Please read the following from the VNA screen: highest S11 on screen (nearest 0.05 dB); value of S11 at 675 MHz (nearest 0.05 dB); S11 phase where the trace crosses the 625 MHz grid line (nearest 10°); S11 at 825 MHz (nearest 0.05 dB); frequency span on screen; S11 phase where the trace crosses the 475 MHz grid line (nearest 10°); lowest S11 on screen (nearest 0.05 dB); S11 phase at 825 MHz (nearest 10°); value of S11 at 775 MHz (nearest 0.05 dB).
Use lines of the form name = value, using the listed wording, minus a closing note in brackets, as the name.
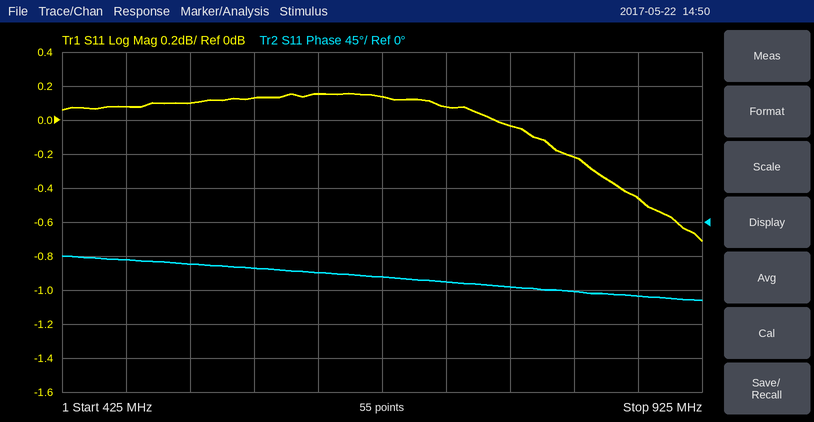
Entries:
highest S11 on screen = 0.15 dB
value of S11 at 675 MHz = 0.15 dB
S11 phase where the trace crosses the 625 MHz grid line = -70°
S11 at 825 MHz = -0.20 dB
frequency span on screen = 500 MHz
S11 phase where the trace crosses the 475 MHz grid line = -50°
lowest S11 on screen = -0.70 dB
S11 phase at 825 MHz = -90°
value of S11 at 775 MHz = -0.05 dB
